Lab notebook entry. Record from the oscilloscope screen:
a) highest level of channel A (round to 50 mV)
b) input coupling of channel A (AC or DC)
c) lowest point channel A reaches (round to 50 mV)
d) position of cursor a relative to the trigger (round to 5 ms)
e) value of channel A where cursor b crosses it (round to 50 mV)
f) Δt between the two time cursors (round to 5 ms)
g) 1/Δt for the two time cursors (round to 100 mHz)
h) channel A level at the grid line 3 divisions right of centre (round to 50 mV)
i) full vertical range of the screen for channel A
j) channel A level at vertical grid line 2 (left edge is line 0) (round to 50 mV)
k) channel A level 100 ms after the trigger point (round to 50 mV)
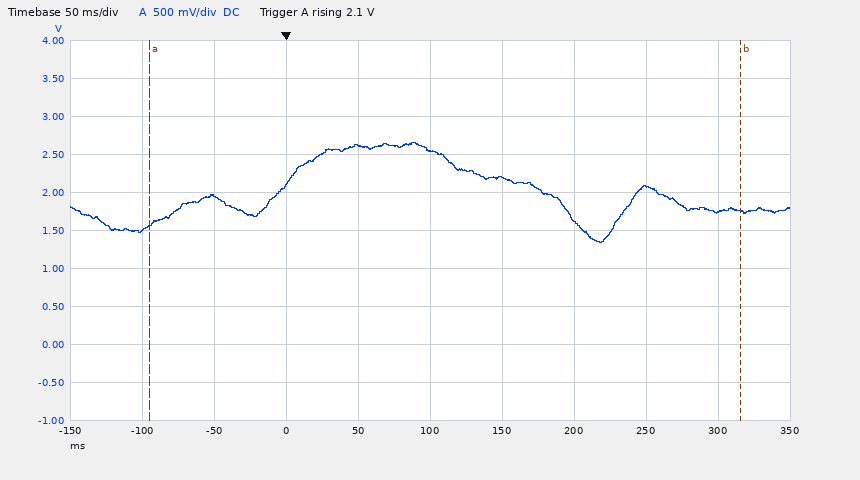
2.65 V
DC
1.35 V
-95 ms
1.75 V
410 ms
2.4 Hz
2.10 V
5 V
1.95 V
2.55 V
